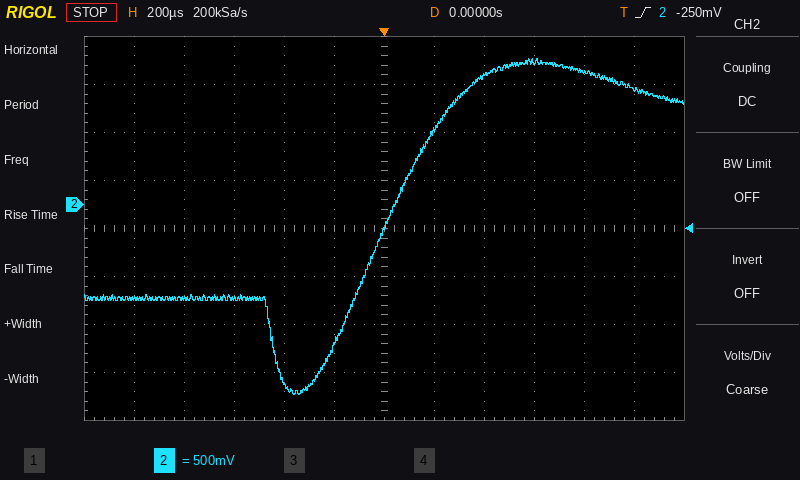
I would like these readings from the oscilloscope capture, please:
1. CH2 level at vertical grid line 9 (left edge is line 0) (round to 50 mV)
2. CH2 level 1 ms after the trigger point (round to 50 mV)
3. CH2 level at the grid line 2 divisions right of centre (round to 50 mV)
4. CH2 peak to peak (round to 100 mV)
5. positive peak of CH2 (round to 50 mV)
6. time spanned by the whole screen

1.50 V
1.20 V
1.35 V
3.50 V
1.50 V
2.4 ms
